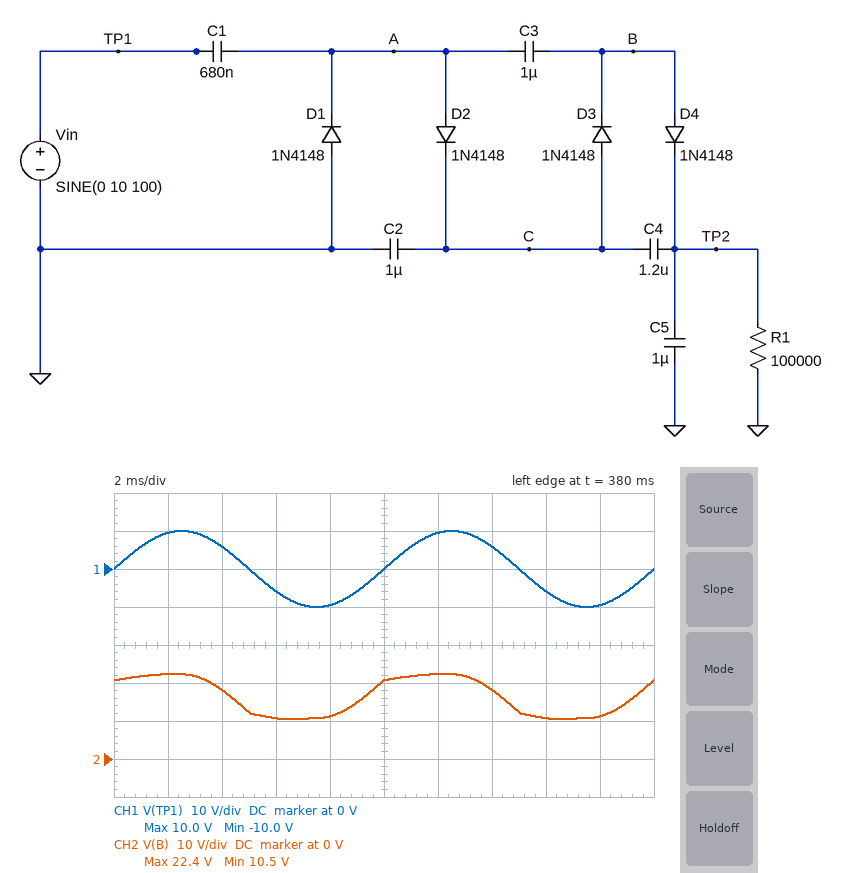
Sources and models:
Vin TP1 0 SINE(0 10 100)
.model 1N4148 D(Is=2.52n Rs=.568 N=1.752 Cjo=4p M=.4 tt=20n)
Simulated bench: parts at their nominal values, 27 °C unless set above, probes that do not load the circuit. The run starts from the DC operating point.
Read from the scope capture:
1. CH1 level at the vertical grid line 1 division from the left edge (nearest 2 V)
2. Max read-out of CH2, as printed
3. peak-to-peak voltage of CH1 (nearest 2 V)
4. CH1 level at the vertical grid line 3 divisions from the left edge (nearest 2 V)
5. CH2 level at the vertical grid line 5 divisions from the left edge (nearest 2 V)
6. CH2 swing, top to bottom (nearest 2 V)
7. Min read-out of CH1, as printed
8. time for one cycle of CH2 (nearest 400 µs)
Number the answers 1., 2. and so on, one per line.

1. 10 V
2. 22.4 V
3. 20 V
4. -6 V
5. 20 V
6. 12 V
7. -10.0 V
8. 10.0 ms
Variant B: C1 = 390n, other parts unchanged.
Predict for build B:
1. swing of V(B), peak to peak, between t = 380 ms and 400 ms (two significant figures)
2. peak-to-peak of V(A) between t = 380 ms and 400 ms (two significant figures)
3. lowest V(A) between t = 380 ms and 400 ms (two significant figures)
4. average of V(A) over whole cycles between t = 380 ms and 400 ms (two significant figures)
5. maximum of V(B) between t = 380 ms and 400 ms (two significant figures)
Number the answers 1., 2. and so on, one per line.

1. 9.6 V
2. 11 V
3. -610 mV
4. 5.0 V
5. 18 V
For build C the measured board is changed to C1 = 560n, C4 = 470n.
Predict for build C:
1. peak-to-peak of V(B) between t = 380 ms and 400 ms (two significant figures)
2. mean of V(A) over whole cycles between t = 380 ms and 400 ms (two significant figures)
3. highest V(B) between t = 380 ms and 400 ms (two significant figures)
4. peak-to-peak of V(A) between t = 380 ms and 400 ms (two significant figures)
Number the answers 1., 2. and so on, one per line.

1. 11 V
2. 5.9 V
3. 21 V
4. 13 V
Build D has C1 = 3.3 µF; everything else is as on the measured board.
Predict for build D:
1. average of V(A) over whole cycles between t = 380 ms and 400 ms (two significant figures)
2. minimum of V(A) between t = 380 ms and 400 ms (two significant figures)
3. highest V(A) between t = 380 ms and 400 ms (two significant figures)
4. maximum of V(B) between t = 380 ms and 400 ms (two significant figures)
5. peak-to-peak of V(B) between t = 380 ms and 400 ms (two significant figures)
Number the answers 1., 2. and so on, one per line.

1. 8.5 V
2. -670 mV
3. 18 V
4. 30 V
5. 16 V
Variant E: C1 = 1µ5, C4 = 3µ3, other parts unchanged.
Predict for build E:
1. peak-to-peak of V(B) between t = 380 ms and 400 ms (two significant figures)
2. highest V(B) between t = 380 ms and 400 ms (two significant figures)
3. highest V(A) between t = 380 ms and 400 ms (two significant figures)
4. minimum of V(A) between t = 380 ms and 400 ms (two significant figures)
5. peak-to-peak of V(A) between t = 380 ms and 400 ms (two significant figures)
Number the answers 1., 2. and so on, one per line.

1. 14 V
2. 27 V
3. 16 V
4. -650 mV
5. 17 V
